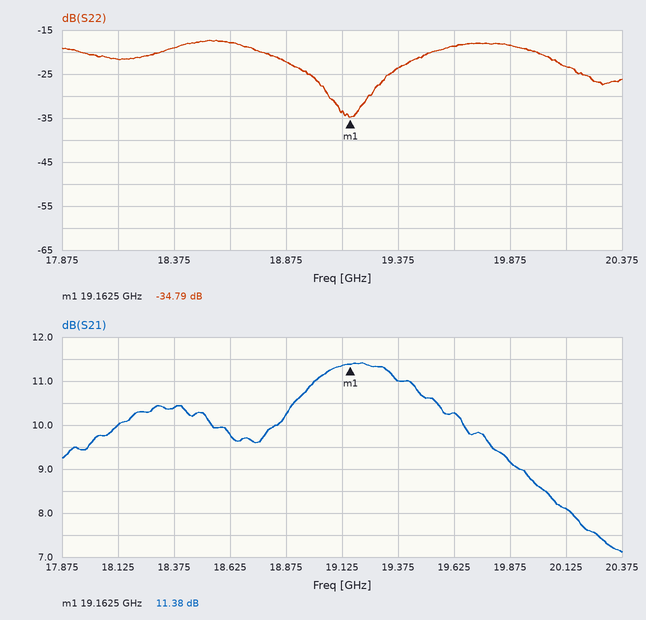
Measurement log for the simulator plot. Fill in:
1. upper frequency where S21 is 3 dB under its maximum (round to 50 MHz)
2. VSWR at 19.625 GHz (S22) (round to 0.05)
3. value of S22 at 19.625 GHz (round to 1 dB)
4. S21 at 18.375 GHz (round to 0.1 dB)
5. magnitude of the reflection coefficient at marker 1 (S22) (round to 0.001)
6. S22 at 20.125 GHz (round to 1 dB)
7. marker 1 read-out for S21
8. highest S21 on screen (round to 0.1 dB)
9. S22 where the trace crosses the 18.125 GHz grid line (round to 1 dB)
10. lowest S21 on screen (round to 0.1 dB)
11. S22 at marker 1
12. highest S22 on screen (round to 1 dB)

20.05 GHz
1.25
-19 dB
10.4 dB
0.018
-23 dB
11.38 dB
11.4 dB
-22 dB
7.1 dB
-34.79 dB
-17 dB
